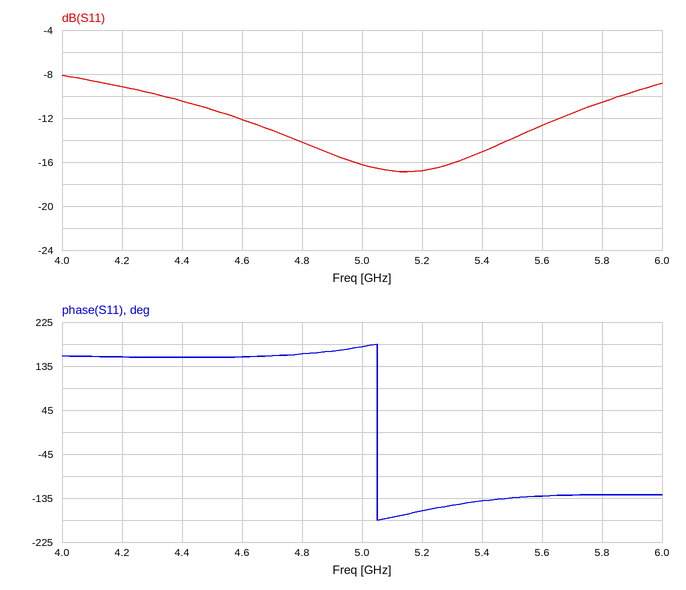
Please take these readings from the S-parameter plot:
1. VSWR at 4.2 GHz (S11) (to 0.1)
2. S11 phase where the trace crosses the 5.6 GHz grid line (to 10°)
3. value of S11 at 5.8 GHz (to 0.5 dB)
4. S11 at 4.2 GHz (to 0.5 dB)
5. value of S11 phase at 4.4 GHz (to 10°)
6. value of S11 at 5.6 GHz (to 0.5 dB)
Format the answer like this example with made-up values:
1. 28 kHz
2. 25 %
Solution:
1. 2.1
2. -130°
3. -10.5 dB
4. -9.0 dB
5. 150°
6. -12.5 dB
